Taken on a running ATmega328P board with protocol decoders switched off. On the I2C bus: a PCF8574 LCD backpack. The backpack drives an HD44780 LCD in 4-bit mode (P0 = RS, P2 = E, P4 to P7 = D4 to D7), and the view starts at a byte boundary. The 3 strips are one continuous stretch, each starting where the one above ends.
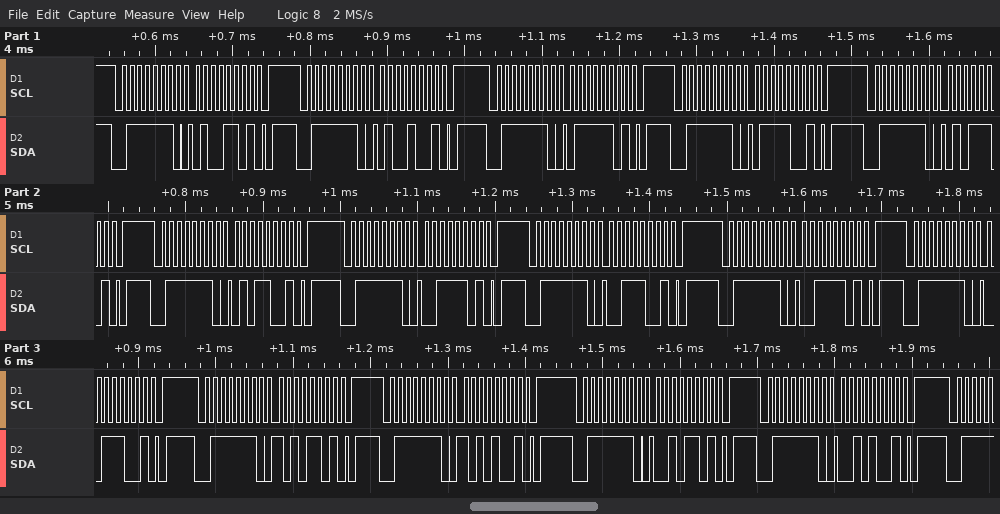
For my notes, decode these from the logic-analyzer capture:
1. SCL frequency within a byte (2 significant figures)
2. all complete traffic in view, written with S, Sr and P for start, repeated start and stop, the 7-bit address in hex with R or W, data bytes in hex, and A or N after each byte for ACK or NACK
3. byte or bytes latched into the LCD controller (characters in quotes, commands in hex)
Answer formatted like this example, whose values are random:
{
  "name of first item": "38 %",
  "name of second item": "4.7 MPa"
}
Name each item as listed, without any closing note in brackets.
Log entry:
{
  "SCL frequency within a byte": "100 kHz",
  "all complete traffic in view, written with S, Sr and P for start, repeated start and stop, the 7-bit address in hex with R or W, data bytes in hex, and A or N after each byte for ACK or NACK": "S 3FW A 4D A P S 3FW A 49 A P S 3FW A 7D A P S 3FW A 79 A P S 3FW A 5D A P S 3FW A 59 A P S 3FW A 3D A P S 3FW A 39 A P S 3FW A 3D A P S 3FW A 39 A P S 3FW A AD A P S 3FW A A9 A P S 3FW A 2D A P S 3FW A 29 A P",
  "byte or bytes latched into the LCD controller": "'G' 'S' ':'"
}
